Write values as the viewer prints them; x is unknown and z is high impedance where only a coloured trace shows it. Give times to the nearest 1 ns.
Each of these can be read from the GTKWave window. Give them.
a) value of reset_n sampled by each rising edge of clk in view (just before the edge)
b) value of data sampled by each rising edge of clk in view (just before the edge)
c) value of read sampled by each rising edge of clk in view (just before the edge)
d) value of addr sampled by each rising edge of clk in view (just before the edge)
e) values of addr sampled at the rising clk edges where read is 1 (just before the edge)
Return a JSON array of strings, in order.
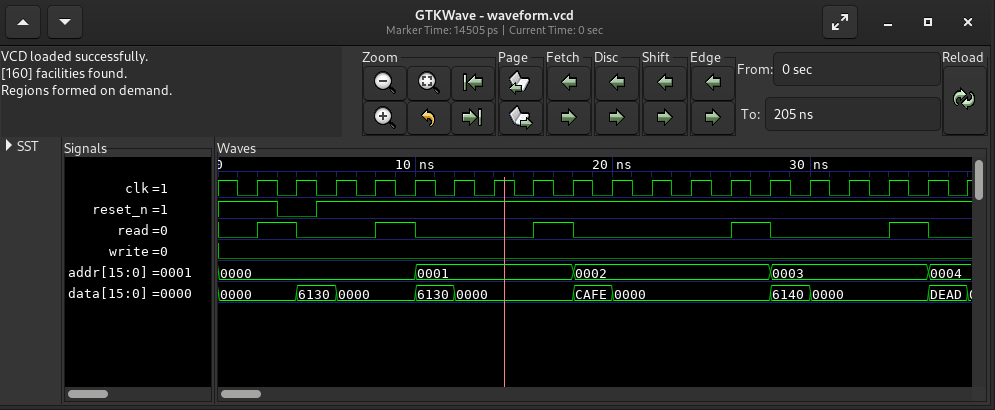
["1 0 1 1 1 1 1 1 1 1 1 1 1 1 1 1 1 1 1", "0000, 0000, 6130, 0000, 0000, 6130, 0000, 0000, 0000, CAFE, 0000, 0000, 0000, 0000, 6140, 0000, 0000, 0000, DEAD", "0 1 0 0 1 0 0 0 1 0 0 0 0 1 0 0 0 1 0", "0000, 0000, 0000, 0000, 0000, 0001, 0001, 0001, 0001, 0002, 0002, 0002, 0002, 0002, 0003, 0003, 0003, 0003, 0004", "0000, 0000, 0001, 0002, 0003"]
